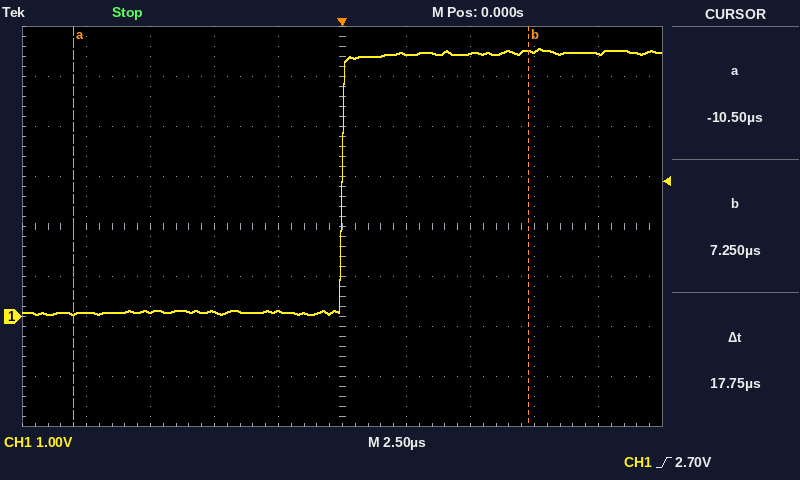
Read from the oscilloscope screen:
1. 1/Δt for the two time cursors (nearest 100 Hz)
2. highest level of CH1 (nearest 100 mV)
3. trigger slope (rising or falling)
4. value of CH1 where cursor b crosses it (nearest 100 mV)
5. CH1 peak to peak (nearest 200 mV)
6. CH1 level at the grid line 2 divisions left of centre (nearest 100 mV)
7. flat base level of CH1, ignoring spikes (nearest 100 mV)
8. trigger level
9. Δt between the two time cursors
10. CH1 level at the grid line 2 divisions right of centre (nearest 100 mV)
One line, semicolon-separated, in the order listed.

56.3 kHz; 5.4 V; rising; 5.3 V; 5.4 V; 100 mV; 100 mV; 2.70 V; 17.75 µs; 5.3 V
